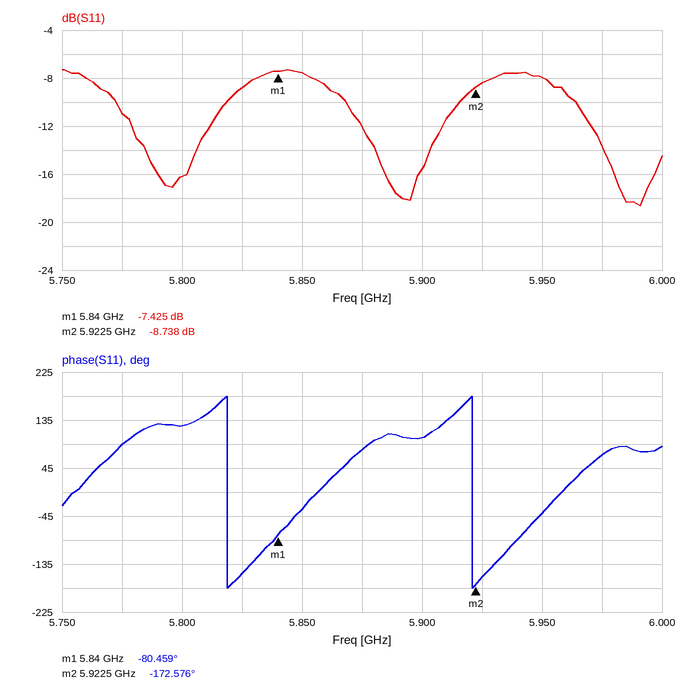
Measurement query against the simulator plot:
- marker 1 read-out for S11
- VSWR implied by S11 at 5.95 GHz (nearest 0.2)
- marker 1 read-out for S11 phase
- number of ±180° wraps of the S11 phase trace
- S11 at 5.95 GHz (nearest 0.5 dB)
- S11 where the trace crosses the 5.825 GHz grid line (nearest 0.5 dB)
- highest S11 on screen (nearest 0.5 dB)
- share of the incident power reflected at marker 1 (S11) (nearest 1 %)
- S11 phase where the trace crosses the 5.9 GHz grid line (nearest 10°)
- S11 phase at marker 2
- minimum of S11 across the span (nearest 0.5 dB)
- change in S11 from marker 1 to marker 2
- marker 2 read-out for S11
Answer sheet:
-7.425 dB
2.4
-80.459°
2
-8.0 dB
-9.0 dB
-7.5 dB
18 %
100°
-172.576°
-18.5 dB
-1.313 dB
-8.738 dB
